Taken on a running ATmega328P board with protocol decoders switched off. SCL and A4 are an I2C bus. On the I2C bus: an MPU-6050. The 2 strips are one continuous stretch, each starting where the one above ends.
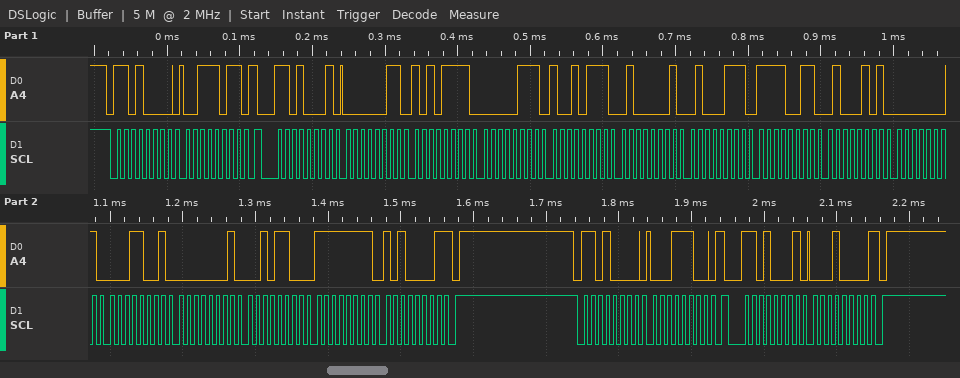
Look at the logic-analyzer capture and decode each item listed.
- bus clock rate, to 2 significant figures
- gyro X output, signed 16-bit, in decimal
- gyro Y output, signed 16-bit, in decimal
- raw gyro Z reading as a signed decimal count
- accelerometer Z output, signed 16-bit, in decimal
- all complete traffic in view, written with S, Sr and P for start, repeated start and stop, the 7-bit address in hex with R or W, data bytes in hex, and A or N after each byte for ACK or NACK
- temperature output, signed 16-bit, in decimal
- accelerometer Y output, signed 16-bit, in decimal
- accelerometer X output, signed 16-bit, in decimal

100 kHz
281
300
-95
16711
S 68W A 3B A Sr 68R A 03 A AF A 07 A 97 A 41 A 47 A F3 A 45 A 01 A 19 A 01 A 2C A FF A A1 N P S 68W A 1C A Sr 68R A 10 N P
-3259
1943
943
